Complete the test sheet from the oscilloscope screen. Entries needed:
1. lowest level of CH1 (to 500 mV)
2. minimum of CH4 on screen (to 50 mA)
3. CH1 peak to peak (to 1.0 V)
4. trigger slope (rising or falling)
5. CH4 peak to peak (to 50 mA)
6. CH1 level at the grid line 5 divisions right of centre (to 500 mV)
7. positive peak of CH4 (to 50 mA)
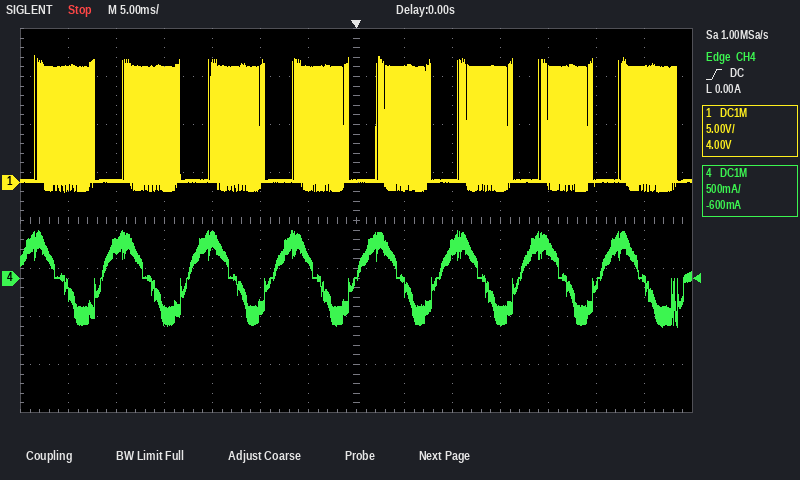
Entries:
-1.0 V
-500 mA
14.0 V
rising
1.00 A
0.0 V
500 mA
